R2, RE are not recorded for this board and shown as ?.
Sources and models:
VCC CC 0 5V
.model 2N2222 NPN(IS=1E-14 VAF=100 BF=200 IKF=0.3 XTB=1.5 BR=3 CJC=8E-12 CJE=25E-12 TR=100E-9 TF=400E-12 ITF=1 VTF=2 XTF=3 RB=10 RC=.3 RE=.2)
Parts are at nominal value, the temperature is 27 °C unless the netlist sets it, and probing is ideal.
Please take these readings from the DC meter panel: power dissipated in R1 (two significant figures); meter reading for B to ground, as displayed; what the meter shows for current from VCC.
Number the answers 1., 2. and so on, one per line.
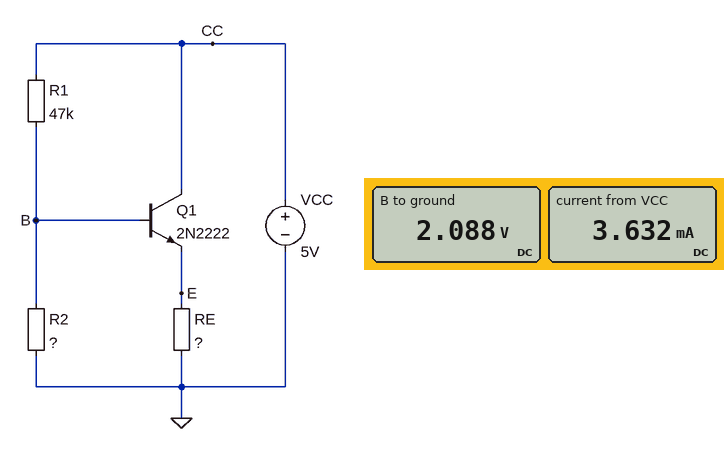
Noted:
1. 180 µW
2. 2.088 V
3. 3.632 mA
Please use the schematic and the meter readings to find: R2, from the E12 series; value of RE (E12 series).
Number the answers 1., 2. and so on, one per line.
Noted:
1. 47 kΩ
2. 390 Ω
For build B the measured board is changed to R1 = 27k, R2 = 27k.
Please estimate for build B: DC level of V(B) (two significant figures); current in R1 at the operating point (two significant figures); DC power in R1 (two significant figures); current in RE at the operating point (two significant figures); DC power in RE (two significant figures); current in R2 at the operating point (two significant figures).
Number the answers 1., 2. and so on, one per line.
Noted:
1. 2.2 V
2. 100 µA
3. 280 µW
4. 4.0 mA
5. 6.1 mW
6. 83 µA
